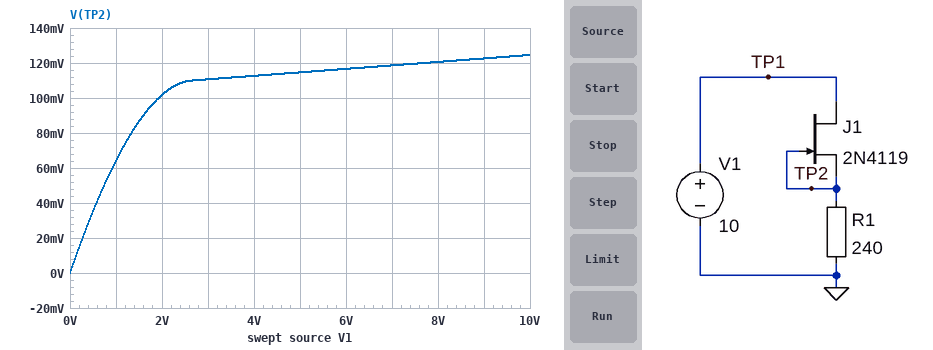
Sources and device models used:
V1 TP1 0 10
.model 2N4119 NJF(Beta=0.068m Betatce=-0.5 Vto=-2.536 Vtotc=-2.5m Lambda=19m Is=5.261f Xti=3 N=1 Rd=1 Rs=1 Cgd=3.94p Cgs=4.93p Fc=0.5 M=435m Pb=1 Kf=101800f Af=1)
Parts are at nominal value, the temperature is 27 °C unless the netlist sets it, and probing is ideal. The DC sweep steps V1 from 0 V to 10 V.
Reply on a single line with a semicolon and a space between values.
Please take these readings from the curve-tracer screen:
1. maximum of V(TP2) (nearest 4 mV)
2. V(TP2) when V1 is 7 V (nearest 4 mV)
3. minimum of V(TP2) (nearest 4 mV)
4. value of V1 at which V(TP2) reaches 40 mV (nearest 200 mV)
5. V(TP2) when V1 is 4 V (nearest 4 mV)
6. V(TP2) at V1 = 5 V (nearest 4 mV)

124 mV; 120 mV; 0 V; 600 mV; 112 mV; 116 mV
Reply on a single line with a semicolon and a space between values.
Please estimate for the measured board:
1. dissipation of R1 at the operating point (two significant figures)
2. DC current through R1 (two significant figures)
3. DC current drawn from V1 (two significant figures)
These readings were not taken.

65 µW; 520 µA; 520 µA
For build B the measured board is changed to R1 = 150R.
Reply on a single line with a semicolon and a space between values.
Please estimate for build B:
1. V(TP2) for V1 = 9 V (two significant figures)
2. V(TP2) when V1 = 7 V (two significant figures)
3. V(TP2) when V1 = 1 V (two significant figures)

77 mV; 74 mV; 41 mV
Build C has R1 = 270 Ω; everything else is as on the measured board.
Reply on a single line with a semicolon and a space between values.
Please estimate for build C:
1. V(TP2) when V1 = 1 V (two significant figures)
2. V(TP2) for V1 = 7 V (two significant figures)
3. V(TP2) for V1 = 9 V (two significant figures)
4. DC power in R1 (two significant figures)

72 mV; 130 mV; 140 mV; 73 µW
